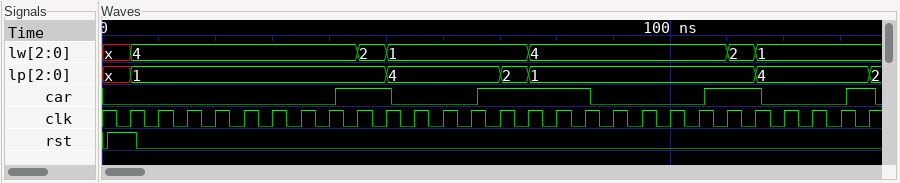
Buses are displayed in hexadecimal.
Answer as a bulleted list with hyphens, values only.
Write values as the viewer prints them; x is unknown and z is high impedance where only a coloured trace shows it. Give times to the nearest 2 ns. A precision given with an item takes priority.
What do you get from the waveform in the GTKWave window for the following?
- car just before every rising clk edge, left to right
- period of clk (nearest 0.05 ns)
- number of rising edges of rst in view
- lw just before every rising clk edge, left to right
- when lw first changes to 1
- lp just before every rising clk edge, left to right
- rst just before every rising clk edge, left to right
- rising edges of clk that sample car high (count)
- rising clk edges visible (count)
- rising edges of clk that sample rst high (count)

- 0 0 0 0 0 0 0 0 1 1 0 0 0 1 1 1 1 0 0 0 0 1 1 0 0 0 1
- 5 ns
- 1
- x, 4, 4, 4, 4, 4, 4, 4, 4, 2, 1, 1, 1, 1, 1, 4, 4, 4, 4, 4, 4, 4, 2, 1, 1, 1, 1
- 50 ns
- x, 1, 1, 1, 1, 1, 1, 1, 1, 1, 4, 4, 4, 4, 2, 1, 1, 1, 1, 1, 1, 1, 1, 4, 4, 4, 4
- 1 0 0 0 0 0 0 0 0 0 0 0 0 0 0 0 0 0 0 0 0 0 0 0 0 0 0
- 9
- 27
- 1
